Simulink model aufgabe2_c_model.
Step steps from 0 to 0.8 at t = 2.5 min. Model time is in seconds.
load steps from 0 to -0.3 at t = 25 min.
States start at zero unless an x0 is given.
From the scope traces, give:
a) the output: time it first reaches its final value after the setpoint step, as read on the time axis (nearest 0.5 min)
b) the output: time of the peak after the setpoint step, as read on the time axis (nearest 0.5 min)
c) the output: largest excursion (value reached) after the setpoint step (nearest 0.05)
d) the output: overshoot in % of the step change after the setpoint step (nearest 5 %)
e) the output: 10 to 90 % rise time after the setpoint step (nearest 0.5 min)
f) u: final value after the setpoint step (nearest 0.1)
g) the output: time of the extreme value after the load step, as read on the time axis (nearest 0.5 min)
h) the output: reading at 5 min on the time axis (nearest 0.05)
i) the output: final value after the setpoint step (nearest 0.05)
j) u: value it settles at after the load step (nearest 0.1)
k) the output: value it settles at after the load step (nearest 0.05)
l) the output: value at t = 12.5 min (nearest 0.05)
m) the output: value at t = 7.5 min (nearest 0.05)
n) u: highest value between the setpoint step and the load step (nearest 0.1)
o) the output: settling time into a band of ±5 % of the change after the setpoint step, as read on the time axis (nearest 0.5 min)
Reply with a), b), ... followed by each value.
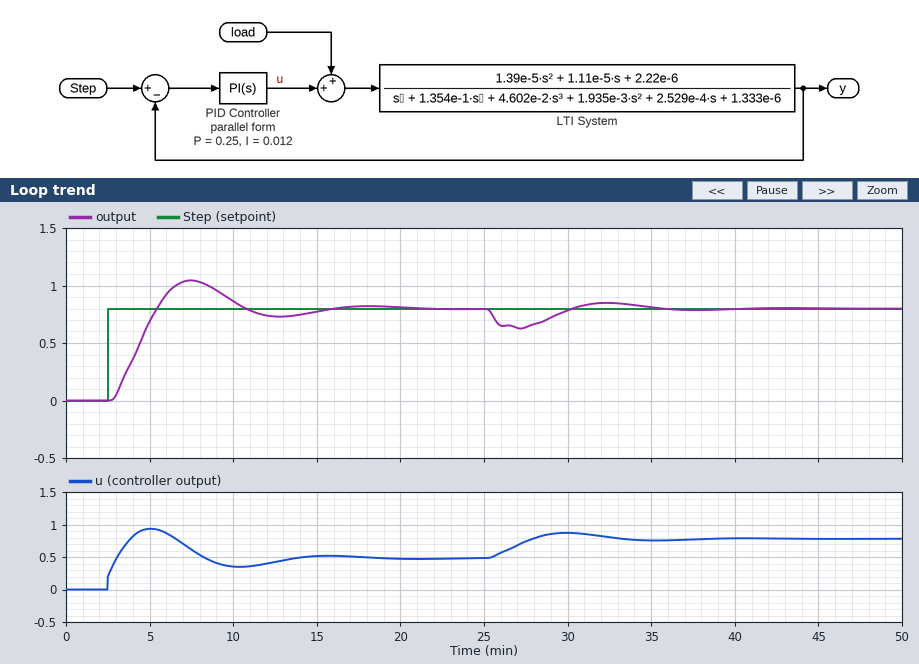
a) 5.5 min
b) 7.5 min
c) 1.05
d) 30 %
e) 2.0 min
f) 0.5
g) 27.0 min
h) 0.70
i) 0.80
j) 0.8
k) 0.80
l) 0.75
m) 1.05
n) 0.9
o) 14.5 min
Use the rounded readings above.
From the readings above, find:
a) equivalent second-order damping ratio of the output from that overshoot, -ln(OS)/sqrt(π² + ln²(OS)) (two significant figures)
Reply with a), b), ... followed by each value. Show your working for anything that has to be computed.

a) ln(0.3) = -1.204; 1.204 / sqrt(9.870 + 1.450) = 0.36
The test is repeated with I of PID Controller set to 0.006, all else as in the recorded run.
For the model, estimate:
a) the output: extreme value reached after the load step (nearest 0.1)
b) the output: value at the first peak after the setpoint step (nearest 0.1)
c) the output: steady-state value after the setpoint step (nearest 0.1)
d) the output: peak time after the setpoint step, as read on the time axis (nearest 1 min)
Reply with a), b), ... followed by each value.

a) 0.6
b) 0.9
c) 0.8
d) 10 min
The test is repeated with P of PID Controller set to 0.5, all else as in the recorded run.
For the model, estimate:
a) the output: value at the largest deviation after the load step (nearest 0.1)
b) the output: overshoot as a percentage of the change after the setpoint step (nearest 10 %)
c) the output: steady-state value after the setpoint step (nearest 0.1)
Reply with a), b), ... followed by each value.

a) 0.6
b) 20 %
c) 0.8
